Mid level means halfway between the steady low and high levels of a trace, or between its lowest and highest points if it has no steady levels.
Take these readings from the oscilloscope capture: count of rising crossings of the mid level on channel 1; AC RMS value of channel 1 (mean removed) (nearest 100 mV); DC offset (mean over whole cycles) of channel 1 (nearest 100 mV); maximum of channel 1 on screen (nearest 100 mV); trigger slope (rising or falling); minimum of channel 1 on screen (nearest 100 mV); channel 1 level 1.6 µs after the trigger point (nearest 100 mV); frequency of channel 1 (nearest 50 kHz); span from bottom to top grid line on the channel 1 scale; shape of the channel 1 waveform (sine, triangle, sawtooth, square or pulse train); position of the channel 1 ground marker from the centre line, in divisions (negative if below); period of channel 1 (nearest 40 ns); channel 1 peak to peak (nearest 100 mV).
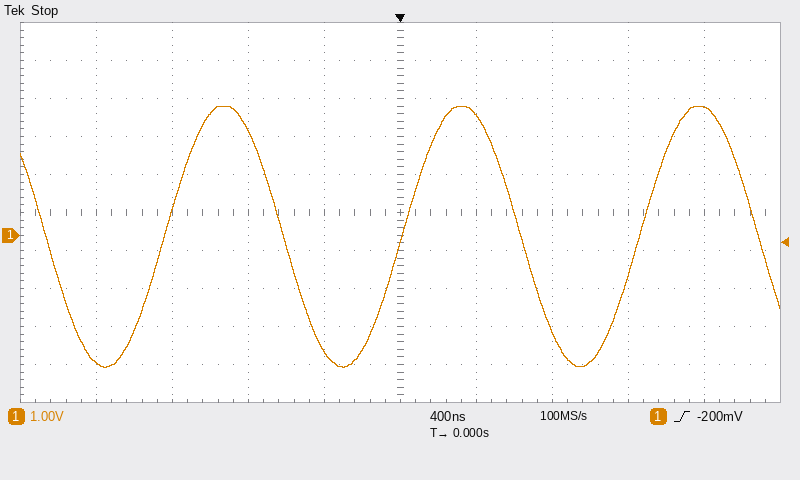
3
2.4 V
0.0 V
3.4 V
rising
-3.5 V
3.4 V
800 kHz
10 V
sine
-0.6 div
1.24 µs
6.9 V
